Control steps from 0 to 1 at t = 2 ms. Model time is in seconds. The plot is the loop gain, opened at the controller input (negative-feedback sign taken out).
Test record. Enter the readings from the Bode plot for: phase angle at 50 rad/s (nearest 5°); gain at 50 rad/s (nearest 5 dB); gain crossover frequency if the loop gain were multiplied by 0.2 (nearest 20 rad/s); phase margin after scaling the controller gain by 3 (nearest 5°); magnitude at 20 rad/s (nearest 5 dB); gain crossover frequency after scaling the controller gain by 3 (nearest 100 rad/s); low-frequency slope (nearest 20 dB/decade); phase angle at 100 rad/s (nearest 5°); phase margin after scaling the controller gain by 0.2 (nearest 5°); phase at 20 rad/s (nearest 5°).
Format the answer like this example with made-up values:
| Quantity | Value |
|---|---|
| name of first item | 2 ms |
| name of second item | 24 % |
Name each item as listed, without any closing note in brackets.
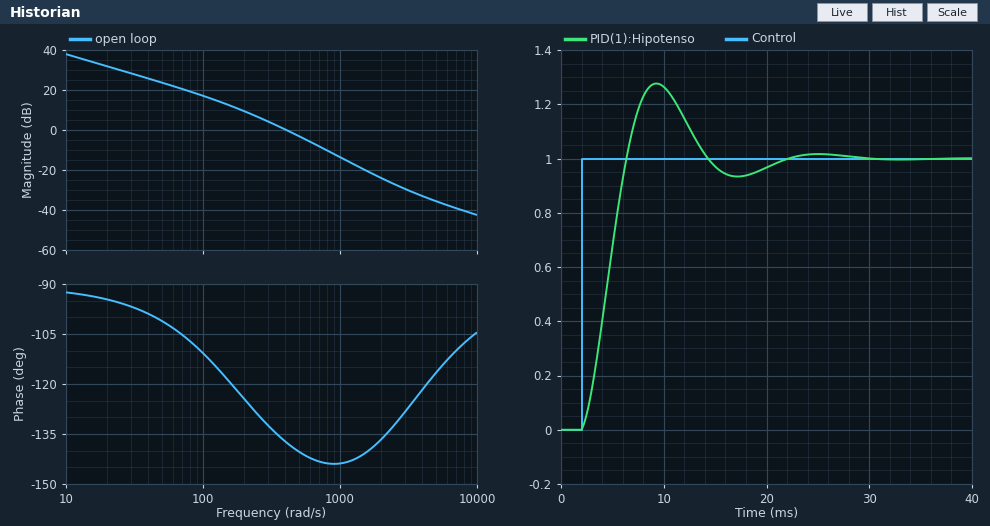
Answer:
| Quantity | Value |
|---|---|
| phase angle at 50 rad/s | -100° |
| gain at 50 rad/s | 25 dB |
| gain crossover frequency if the loop gain were multiplied by 0.2 | 140 rad/s |
| phase margin after scaling the controller gain by 3 | 35° |
| magnitude at 20 rad/s | 30 dB |
| gain crossover frequency after scaling the controller gain by 3 | 800 rad/s |
| low-frequency slope | -20 dB/decade |
| phase angle at 100 rad/s | -110° |
| phase margin after scaling the controller gain by 0.2 | 65° |
| phase at 20 rad/s | -95° |
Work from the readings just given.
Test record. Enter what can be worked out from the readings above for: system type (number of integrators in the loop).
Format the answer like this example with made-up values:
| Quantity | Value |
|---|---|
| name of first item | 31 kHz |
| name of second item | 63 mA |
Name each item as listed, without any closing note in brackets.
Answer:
| Quantity | Value |
|---|---|
| system type | 1 |
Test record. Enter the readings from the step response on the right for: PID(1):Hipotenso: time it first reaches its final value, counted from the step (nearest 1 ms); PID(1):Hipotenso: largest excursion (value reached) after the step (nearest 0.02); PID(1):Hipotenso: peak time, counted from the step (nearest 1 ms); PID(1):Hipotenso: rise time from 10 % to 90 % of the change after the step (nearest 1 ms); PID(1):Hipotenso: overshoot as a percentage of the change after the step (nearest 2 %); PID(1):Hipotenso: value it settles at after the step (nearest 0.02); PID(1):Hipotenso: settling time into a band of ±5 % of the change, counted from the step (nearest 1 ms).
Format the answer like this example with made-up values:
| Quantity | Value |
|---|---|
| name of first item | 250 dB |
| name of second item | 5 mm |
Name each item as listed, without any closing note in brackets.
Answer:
| Quantity | Value |
|---|---|
| PID(1):Hipotenso: time it first reaches its final value, counted from the step | 4 ms |
| PID(1):Hipotenso: largest excursion (value reached) after the step | 1.28 |
| PID(1):Hipotenso: peak time, counted from the step | 7 ms |
| PID(1):Hipotenso: rise time from 10 % to 90 % of the change after the step | 3 ms |
| PID(1):Hipotenso: overshoot as a percentage of the change after the step | 28 % |
| PID(1):Hipotenso: value it settles at after the step | 1.00 |
| PID(1):Hipotenso: settling time into a band of ±5 % of the change, counted from the step | 17 ms |
